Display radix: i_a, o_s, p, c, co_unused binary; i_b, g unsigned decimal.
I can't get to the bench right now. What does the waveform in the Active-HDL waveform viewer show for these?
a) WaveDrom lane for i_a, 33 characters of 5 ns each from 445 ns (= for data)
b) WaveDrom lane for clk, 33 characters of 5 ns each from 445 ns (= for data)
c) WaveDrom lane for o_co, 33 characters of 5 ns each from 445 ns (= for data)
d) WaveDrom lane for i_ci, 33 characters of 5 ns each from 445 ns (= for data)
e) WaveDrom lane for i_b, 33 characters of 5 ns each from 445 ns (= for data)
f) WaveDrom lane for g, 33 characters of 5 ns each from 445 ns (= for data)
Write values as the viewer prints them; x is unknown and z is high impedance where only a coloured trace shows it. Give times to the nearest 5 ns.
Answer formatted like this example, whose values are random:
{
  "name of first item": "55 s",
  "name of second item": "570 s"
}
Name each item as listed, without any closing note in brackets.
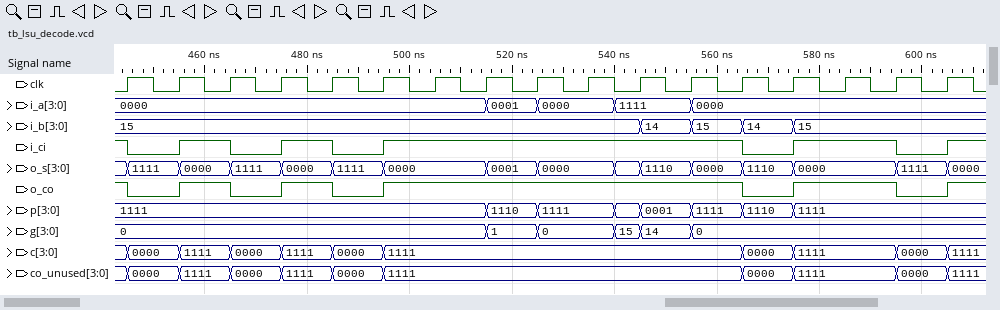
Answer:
{
  "WaveDrom lane for i_a, 33 characters of 5 ns each from 445 ns": "{name: 'i_a', wave: '=.............=.=..=..=..........', data: '0000 0001 0000 1111 0000'}",
  "WaveDrom lane for clk, 33 characters of 5 ns each from 445 ns": "{name: 'clk', wave: '101010101010101010101010101010101'}",
  "WaveDrom lane for o_co, 33 characters of 5 ns each from 445 ns": "{name: 'o_co', wave: '0.1.0.1.0.1.............0.1...0.1'}",
  "WaveDrom lane for i_ci, 33 characters of 5 ns each from 445 ns": "{name: 'i_ci', wave: '0.1.0.1.0.1.............0.1...0.1'}",
  "WaveDrom lane for i_b, 33 characters of 5 ns each from 445 ns": "{name: 'i_b', wave: '=...................=.=.=.=......', data: '15 14 15 14 15'}",
  "WaveDrom lane for g, 33 characters of 5 ns each from 445 ns": "{name: 'g', wave: '=.............=.=..==.=..........', data: '0 1 0 15 14 0'}"
}
